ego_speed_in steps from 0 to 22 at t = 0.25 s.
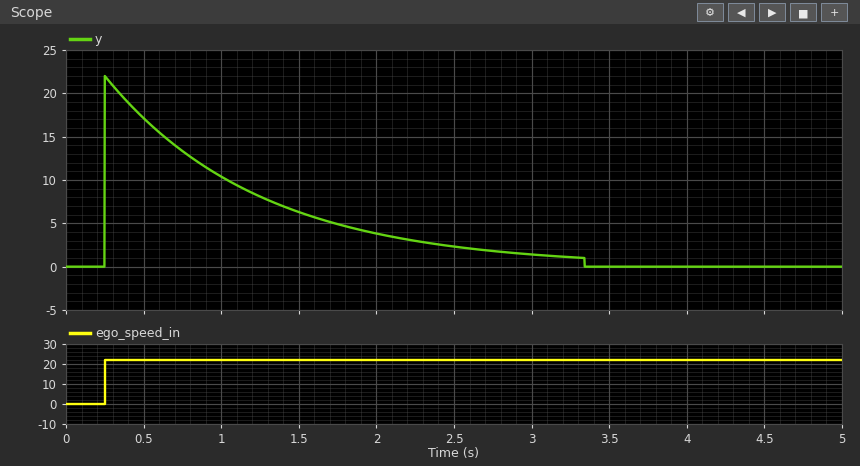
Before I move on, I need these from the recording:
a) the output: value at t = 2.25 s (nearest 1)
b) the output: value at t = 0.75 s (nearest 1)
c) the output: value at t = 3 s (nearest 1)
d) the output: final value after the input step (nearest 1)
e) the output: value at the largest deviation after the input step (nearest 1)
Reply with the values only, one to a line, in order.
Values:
3
13
1
0
22
